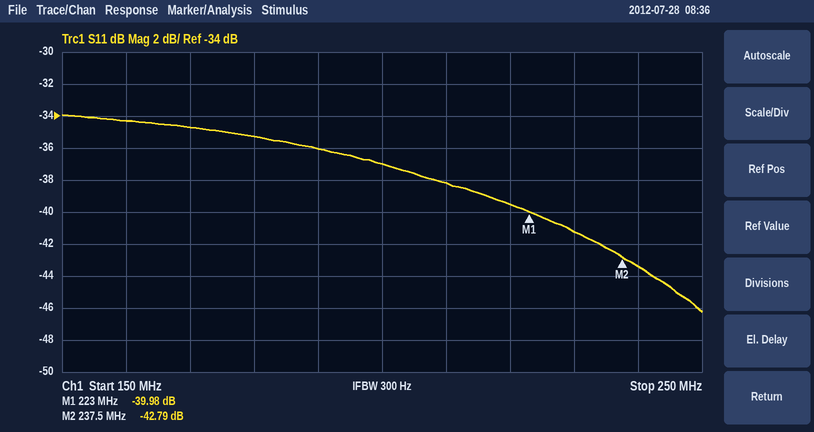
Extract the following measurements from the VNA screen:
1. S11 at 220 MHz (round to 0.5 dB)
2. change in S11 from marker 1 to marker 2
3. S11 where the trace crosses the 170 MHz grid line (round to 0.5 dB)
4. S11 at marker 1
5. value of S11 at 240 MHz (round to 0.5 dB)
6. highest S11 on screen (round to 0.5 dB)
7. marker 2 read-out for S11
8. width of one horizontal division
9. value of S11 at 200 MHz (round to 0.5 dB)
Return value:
-39.5 dB
-2.81 dB
-34.5 dB
-39.98 dB
-43.5 dB
-34.0 dB
-42.79 dB
10 MHz
-37.0 dB
